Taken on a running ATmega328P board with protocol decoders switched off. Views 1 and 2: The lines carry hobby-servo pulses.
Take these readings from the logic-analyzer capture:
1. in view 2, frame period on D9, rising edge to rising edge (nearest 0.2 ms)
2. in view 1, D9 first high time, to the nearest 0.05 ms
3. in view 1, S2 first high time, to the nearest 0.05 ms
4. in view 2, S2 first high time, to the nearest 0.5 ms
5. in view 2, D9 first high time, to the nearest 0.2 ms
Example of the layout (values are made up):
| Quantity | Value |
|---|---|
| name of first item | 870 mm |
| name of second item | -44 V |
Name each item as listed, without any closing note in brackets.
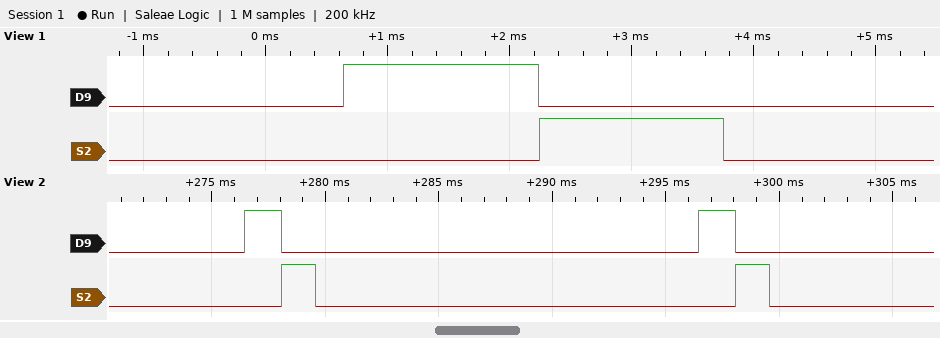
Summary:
| Quantity | Value |
|---|---|
| in view 2, frame period on D9, rising edge to rising edge | 20.0 ms |
| in view 1, D9 first high time, to the nearest 0.05 ms | 1.60 ms |
| in view 1, S2 first high time, to the nearest 0.05 ms | 1.50 ms |
| in view 2, S2 first high time, to the nearest 0.5 ms | 1.5 ms |
| in view 2, D9 first high time, to the nearest 0.2 ms | 1.6 ms |
